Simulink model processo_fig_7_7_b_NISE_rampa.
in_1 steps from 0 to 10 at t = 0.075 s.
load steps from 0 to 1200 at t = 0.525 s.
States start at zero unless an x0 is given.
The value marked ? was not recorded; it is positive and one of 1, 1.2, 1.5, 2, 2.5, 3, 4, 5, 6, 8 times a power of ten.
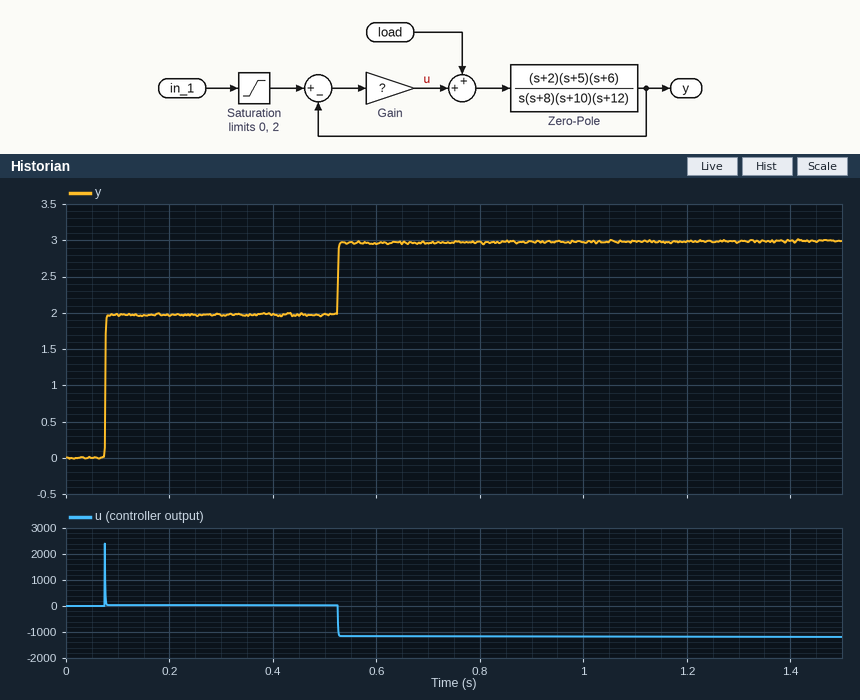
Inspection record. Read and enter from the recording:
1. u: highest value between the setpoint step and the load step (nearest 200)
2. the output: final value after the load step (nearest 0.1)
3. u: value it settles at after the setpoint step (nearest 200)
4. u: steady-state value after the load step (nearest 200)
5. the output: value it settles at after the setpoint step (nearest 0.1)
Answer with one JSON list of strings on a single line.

["2400", "3.0", "0", "-1200", "2.0"]
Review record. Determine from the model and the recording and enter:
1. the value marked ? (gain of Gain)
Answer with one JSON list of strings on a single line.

["1200"]
